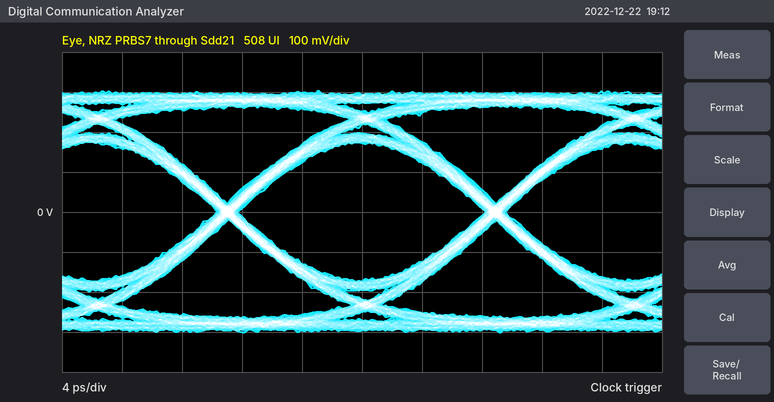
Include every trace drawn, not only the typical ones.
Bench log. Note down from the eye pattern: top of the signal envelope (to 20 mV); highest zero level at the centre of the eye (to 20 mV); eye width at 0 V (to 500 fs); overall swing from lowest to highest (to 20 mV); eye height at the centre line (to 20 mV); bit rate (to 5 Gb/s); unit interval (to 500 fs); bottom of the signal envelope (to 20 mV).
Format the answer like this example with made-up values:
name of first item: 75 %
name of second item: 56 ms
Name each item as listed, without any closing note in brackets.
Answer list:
top of the signal envelope: 300 mV
highest zero level at the centre of the eye: -180 mV
eye width at 0 V: 16.5 ps
overall swing from lowest to highest: 600 mV
eye height at the centre line: 340 mV
bit rate: 55 Gb/s
unit interval: 18.0 ps
bottom of the signal envelope: -300 mV
